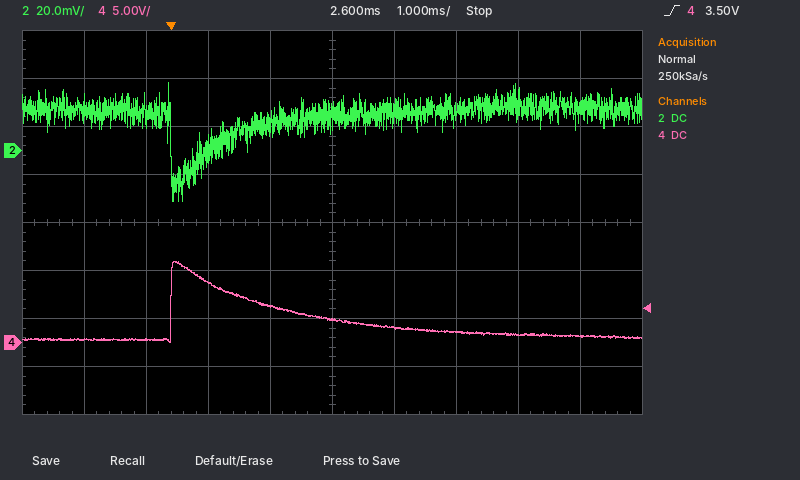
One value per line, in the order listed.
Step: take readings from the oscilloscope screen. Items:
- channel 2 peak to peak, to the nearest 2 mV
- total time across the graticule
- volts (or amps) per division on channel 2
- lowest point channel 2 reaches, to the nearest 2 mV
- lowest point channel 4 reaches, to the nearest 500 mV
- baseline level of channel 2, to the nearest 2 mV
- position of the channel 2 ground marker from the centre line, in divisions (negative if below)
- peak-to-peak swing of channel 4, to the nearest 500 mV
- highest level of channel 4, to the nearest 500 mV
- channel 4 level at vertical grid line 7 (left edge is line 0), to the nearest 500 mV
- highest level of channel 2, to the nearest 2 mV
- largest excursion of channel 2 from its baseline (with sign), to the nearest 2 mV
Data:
50 mV
10 ms
20 mV
-22 mV
0.0 V
16 mV
+1.5 div
8.5 V
8.5 V
1.0 V
28 mV
-38 mV
